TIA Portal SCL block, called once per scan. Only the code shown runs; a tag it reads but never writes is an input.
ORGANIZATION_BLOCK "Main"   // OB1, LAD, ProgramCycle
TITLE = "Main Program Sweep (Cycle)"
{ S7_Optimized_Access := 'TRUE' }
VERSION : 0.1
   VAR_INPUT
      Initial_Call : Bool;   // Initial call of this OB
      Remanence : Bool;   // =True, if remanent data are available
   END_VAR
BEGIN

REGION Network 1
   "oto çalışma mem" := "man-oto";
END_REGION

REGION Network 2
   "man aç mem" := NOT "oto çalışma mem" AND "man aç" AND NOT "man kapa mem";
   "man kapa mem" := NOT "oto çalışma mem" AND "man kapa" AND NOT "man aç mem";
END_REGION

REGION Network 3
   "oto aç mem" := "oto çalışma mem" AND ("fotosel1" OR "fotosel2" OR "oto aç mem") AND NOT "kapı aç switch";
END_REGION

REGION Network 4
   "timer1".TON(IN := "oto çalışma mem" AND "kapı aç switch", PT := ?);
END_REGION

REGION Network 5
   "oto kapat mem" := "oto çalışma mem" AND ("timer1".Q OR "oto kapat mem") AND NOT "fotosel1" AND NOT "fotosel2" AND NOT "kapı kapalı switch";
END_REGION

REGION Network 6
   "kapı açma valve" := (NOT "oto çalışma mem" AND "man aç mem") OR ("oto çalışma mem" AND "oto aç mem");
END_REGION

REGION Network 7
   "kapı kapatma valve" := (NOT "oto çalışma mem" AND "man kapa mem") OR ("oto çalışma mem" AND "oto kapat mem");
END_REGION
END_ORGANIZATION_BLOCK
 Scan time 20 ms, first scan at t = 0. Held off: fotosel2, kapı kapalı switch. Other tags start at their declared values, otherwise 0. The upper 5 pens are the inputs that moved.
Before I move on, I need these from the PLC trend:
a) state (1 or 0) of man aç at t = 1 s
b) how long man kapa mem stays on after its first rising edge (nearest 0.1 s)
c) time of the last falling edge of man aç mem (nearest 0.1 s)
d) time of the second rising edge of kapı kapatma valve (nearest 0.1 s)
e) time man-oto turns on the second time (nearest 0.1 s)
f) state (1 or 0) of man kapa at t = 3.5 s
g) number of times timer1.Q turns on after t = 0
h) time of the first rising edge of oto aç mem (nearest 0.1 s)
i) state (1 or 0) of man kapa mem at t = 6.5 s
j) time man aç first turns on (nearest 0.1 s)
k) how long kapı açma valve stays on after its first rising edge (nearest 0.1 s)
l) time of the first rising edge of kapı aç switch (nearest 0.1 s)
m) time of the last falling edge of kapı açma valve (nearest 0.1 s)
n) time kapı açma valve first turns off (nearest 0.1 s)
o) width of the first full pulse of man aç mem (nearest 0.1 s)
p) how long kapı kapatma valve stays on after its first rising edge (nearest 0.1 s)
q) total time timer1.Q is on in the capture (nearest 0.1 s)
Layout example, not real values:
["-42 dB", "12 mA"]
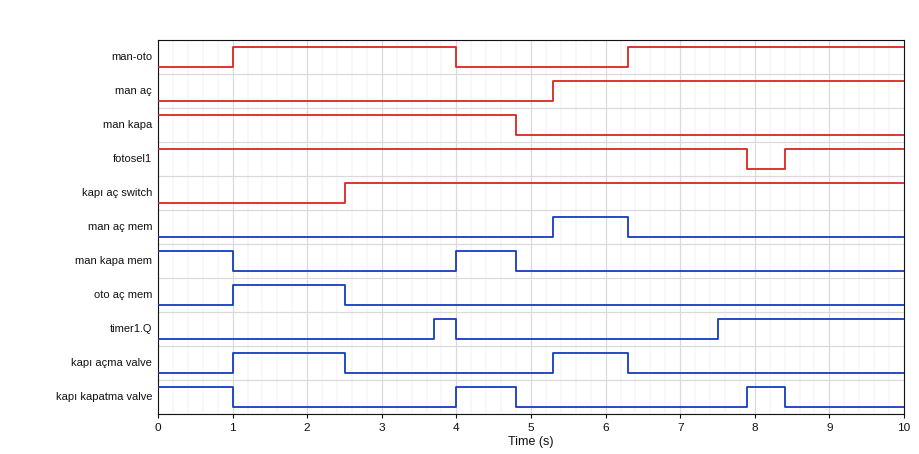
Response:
["0", "0.8 s", "6.3 s", "7.9 s", "6.3 s", "1", "2", "1.0 s", "0", "5.3 s", "1.5 s", "2.5 s", "6.3 s", "2.5 s", "1.0 s", "0.8 s", "2.8 s"]
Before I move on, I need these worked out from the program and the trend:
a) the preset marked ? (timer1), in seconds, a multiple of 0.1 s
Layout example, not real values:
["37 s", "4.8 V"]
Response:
["1.2 s"]
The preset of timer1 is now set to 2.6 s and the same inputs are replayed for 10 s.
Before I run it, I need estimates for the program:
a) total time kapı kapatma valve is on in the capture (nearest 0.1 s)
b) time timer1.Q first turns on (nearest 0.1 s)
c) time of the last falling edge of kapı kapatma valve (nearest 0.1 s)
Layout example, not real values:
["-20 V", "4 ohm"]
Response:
["1.8 s", "8.9 s", "4.8 s"]
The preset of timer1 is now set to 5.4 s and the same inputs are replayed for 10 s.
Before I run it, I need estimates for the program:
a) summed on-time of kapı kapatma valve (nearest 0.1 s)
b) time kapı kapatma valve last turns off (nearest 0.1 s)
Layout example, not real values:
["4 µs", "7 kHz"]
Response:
["1.8 s", "4.8 s"]
